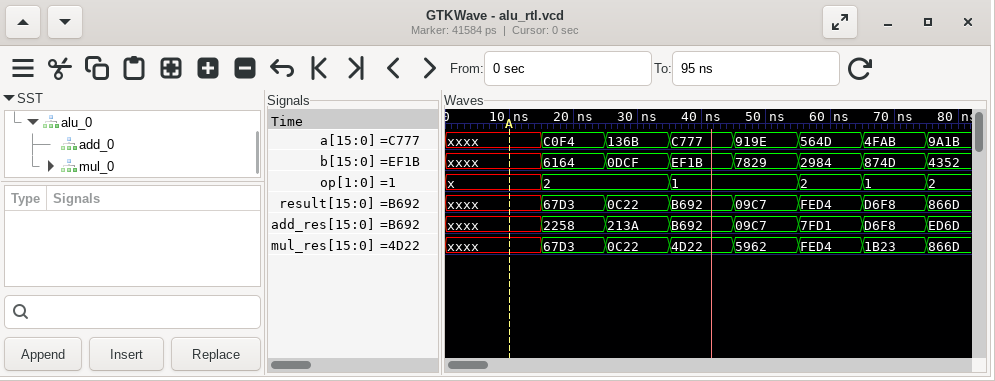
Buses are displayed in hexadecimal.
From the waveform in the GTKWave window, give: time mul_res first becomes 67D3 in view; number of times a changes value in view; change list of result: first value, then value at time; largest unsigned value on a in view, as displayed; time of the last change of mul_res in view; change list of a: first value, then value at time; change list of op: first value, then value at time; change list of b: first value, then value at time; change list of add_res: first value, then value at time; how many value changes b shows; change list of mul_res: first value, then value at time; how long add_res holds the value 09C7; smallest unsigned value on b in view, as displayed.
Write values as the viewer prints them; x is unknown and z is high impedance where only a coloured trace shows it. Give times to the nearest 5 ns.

15 ns
7
xxxx, 67D3 at 15 ns, 0C22 at 25 ns, B692 at 35 ns, 09C7 at 45 ns, FED4 at 55 ns, D6F8 at 65 ns, 866D at 75 ns
C777
75 ns
xxxx, C0F4 at 15 ns, 136B at 25 ns, C777 at 35 ns, 919E at 45 ns, 564D at 55 ns, 4FAB at 65 ns, 9A1B at 75 ns
x, 2 at 15 ns, 1 at 35 ns, 2 at 55 ns, 1 at 65 ns, 2 at 75 ns
xxxx, 6164 at 15 ns, 0DCF at 25 ns, EF1B at 35 ns, 7829 at 45 ns, 2984 at 55 ns, 874D at 65 ns, 4352 at 75 ns
xxxx, 2258 at 15 ns, 213A at 25 ns, B692 at 35 ns, 09C7 at 45 ns, 7FD1 at 55 ns, D6F8 at 65 ns, ED6D at 75 ns
7
xxxx, 67D3 at 15 ns, 0C22 at 25 ns, 4D22 at 35 ns, 5962 at 45 ns, FED4 at 55 ns, 1B23 at 65 ns, 866D at 75 ns
10 ns
0DCF
